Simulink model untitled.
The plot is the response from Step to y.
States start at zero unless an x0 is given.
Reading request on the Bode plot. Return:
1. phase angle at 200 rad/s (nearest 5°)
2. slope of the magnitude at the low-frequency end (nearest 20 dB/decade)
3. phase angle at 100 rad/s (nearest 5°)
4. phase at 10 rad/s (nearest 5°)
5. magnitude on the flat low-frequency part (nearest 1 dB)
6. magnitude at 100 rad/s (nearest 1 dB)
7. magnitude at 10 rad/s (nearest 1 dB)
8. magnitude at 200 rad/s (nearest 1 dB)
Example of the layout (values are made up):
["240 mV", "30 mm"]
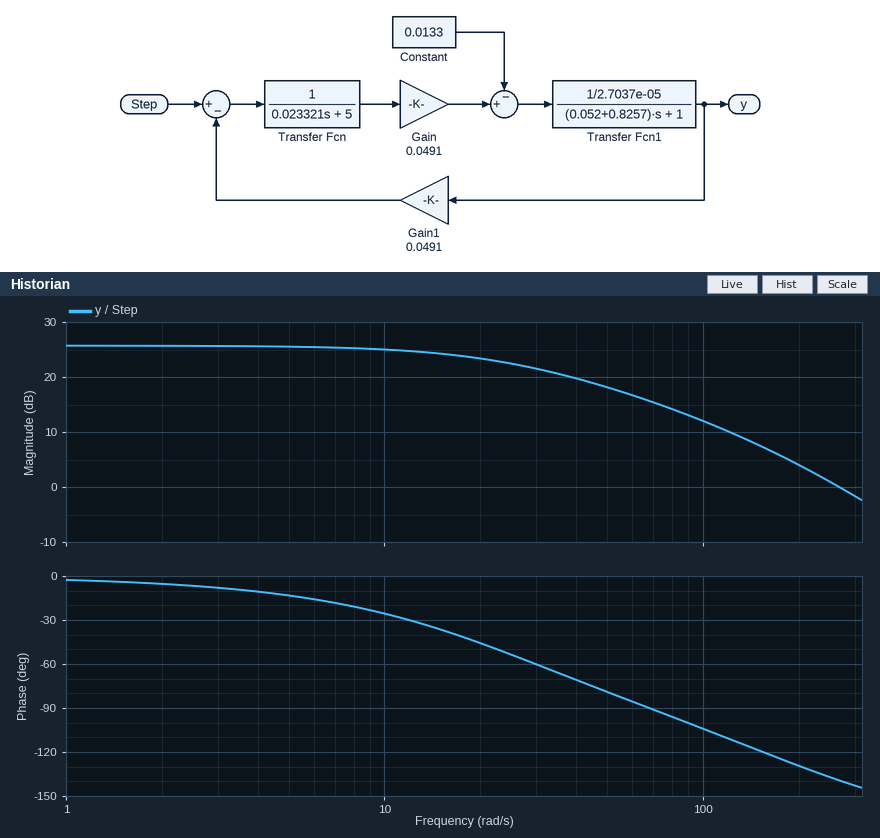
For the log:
["-130°", "0 dB/decade", "-105°", "-25°", "26 dB", "12 dB", "25 dB", "4 dB"]
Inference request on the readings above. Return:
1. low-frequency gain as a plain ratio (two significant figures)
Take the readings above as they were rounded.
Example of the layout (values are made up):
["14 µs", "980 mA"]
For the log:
["20"]
